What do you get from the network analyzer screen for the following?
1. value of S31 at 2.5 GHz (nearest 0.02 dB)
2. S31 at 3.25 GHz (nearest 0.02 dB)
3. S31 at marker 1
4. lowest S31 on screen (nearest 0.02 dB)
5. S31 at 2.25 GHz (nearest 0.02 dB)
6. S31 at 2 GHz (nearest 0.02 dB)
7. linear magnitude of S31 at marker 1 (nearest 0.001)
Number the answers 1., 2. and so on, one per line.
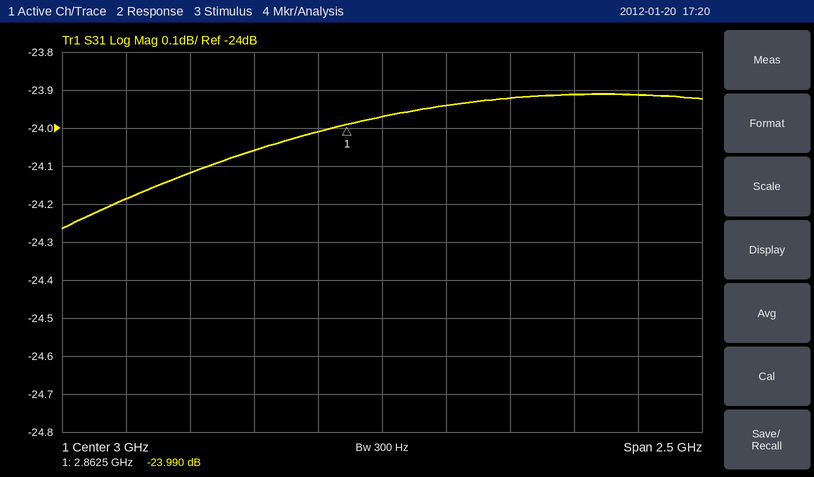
1. -24.06 dB
2. -23.94 dB
3. -23.990 dB
4. -24.26 dB
5. -24.12 dB
6. -24.18 dB
7. 0.063
